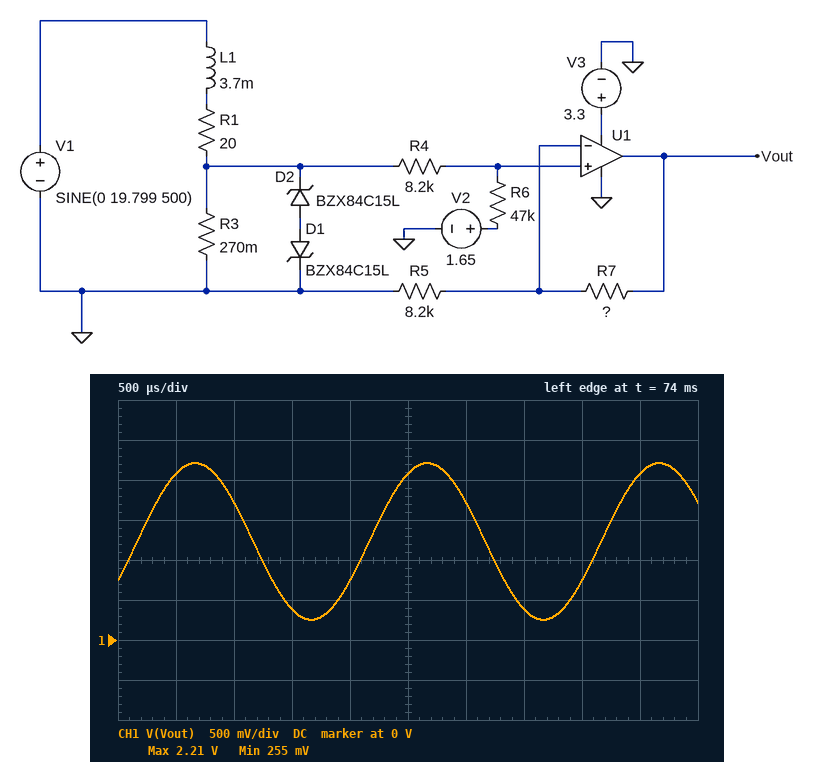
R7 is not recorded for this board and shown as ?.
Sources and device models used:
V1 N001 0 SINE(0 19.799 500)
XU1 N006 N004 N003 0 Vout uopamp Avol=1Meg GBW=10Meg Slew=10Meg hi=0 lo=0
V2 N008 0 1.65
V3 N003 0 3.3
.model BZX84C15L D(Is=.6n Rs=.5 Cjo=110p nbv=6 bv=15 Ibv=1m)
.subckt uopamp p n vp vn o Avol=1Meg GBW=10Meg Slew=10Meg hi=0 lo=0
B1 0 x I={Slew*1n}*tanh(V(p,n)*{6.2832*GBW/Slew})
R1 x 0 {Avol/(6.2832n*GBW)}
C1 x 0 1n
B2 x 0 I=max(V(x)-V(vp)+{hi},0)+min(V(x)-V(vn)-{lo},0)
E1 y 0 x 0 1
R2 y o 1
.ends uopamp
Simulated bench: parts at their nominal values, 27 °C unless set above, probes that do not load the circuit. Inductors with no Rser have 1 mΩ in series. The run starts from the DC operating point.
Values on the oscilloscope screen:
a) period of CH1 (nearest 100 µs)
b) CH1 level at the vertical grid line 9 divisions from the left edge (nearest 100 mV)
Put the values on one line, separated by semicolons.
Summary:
2.0 ms; 2.1 V
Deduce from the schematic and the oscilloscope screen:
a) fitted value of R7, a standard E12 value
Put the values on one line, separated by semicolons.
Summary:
33 kΩ
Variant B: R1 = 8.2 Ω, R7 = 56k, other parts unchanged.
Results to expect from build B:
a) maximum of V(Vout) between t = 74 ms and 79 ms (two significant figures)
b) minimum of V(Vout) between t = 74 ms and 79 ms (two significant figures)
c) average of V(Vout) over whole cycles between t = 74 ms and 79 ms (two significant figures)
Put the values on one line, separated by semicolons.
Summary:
3.3 V; -4.2 mV; 1.8 V
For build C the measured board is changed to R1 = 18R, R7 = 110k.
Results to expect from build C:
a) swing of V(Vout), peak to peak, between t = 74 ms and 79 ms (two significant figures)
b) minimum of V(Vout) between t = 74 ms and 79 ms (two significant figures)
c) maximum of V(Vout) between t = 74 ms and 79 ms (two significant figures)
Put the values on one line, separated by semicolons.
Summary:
2.8 V; 500 mV; 3.3 V
